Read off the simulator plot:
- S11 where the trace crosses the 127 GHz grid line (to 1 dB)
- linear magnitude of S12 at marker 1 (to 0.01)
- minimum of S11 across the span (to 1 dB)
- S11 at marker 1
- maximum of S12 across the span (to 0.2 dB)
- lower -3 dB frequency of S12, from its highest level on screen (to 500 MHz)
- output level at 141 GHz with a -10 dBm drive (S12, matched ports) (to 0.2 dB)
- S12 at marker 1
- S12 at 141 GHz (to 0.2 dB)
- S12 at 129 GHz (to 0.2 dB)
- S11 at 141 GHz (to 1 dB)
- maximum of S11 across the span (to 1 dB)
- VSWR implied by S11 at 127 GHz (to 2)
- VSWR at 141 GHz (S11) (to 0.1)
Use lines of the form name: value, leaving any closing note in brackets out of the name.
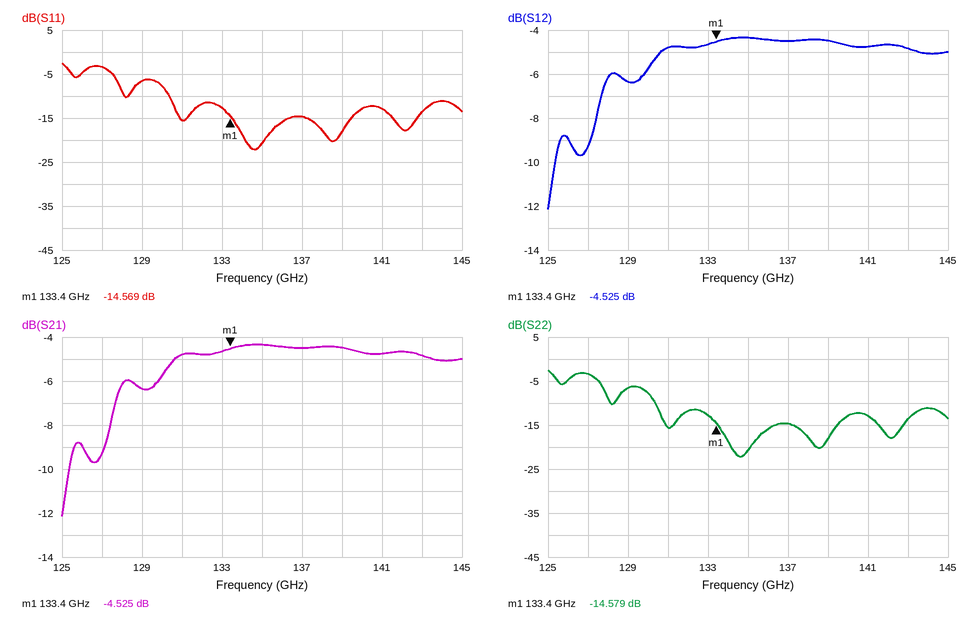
S11 where the trace crosses the 127 GHz grid line: -3 dB
linear magnitude of S12 at marker 1: 0.59
minimum of S11 across the span: -22 dB
S11 at marker 1: -14.569 dB
maximum of S12 across the span: -4.4 dB
lower -3 dB frequency of S12, from its highest level on screen: 127.5 GHz
output level at 141 GHz with a -10 dBm drive (S12, matched ports): -14.8 dBm
S12 at marker 1: -4.525 dB
S12 at 141 GHz: -4.8 dB
S12 at 129 GHz: -6.4 dB
S11 at 141 GHz: -13 dB
maximum of S11 across the span: -3 dB
VSWR implied by S11 at 127 GHz: 6
VSWR at 141 GHz (S11): 1.6
